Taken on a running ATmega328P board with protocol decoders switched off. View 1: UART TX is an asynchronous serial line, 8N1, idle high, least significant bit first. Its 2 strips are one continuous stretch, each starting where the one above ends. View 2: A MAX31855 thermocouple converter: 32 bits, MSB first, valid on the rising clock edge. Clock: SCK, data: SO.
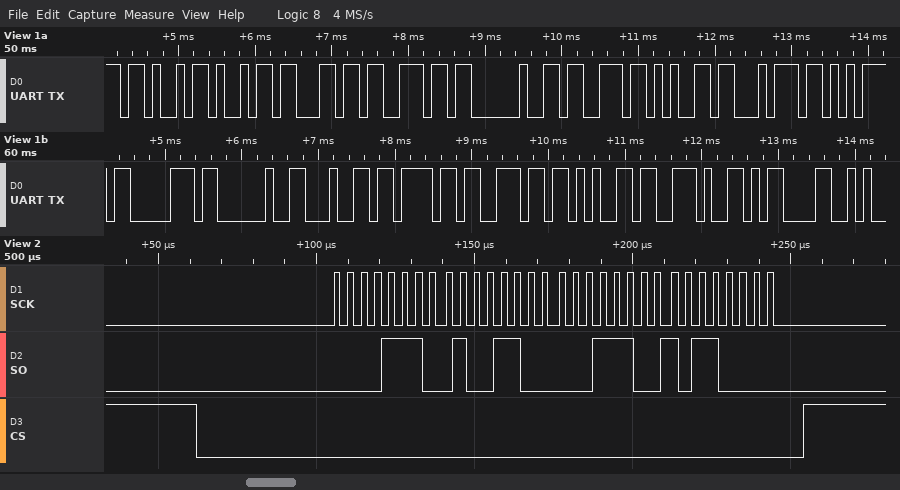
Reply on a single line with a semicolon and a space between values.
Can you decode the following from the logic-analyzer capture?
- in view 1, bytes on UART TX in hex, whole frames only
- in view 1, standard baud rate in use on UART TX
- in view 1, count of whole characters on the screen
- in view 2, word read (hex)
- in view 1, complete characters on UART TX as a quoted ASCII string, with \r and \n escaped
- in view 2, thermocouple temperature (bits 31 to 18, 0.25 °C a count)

4B 69 6C 6E 20 73 65 74 75 70 20 64 6F 6E 65 2E 0D; 9600 baud; 17; 0x0E4C1CB0; "Kiln setup done.\r"; 228.75 °C
